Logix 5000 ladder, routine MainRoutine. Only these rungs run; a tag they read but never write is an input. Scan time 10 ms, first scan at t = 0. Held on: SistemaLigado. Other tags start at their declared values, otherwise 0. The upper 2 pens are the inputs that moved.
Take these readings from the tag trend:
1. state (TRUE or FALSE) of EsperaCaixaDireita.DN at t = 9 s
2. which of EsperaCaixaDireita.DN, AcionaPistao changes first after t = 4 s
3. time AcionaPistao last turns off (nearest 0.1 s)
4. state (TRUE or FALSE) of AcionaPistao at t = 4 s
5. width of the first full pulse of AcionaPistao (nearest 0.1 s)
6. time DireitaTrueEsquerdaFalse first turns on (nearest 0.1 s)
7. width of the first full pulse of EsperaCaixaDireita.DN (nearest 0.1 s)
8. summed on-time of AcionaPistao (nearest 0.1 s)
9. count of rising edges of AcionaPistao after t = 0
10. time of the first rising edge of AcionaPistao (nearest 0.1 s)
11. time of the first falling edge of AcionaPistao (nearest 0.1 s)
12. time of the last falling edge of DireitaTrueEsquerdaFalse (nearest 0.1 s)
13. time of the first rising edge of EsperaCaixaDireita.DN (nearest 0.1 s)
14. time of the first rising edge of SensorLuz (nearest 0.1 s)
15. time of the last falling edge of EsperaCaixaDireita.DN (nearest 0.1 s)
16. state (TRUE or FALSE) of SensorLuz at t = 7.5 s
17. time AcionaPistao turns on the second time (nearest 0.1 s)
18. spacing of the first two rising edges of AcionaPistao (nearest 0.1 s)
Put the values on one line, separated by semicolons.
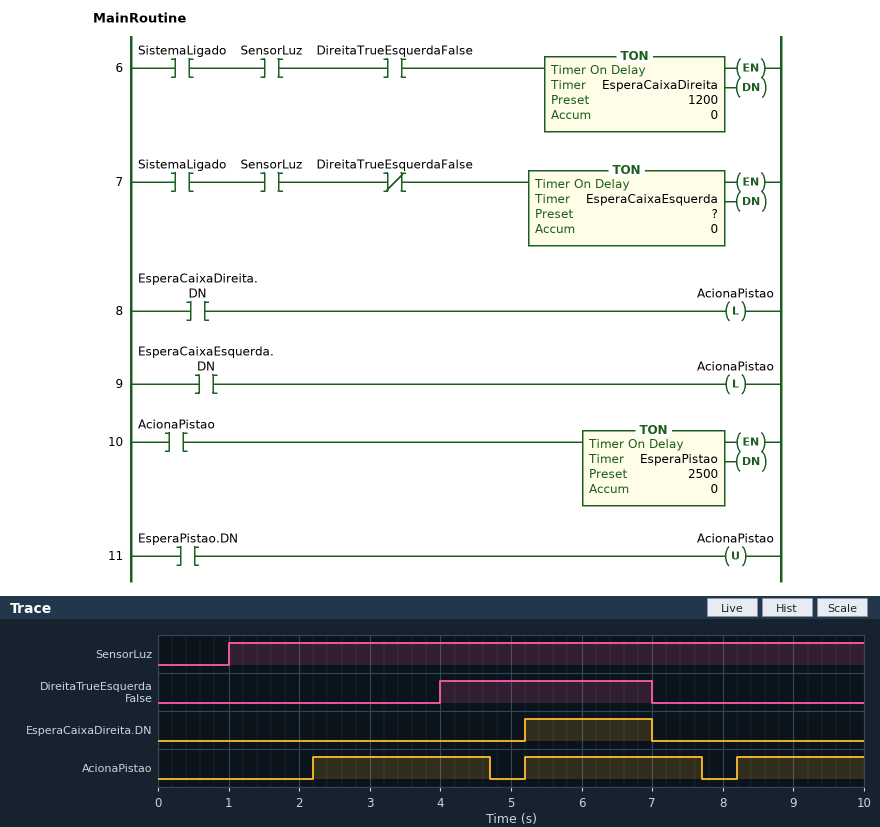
FALSE; AcionaPistao; 7.7 s; TRUE; 2.5 s; 4.0 s; 1.8 s; 6.8 s; 3; 2.2 s; 4.7 s; 7.0 s; 5.2 s; 1.0 s; 7.0 s; TRUE; 5.2 s; 3.0 s
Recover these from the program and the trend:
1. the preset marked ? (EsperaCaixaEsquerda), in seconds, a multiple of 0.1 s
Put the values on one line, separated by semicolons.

1.2 s
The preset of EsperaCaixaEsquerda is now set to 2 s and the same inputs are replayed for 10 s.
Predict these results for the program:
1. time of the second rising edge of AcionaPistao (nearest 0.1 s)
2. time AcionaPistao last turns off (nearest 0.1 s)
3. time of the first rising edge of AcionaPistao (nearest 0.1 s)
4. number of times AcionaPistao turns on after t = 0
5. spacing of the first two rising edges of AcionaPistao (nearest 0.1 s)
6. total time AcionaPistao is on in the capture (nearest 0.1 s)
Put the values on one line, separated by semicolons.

9.0 s; 5.5 s; 3.0 s; 2; 6.0 s; 3.5 s
